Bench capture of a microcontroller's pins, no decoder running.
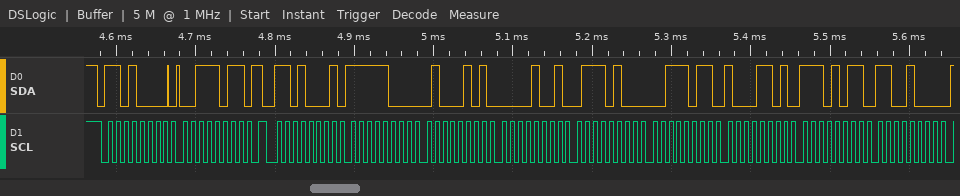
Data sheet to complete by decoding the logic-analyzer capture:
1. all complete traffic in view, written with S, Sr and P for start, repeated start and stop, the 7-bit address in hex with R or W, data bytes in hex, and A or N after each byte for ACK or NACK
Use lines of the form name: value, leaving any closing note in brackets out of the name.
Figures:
all complete traffic in view, written with S, Sr and P for start, repeated start and stop, the 7-bit address in hex with R or W, data bytes in hex, and A or N after each byte for ACK or NACK: S 68W A 3B A Sr 68R A F8 A 45 A 09 A 74 A 3B A 8D A EB A C8 A
